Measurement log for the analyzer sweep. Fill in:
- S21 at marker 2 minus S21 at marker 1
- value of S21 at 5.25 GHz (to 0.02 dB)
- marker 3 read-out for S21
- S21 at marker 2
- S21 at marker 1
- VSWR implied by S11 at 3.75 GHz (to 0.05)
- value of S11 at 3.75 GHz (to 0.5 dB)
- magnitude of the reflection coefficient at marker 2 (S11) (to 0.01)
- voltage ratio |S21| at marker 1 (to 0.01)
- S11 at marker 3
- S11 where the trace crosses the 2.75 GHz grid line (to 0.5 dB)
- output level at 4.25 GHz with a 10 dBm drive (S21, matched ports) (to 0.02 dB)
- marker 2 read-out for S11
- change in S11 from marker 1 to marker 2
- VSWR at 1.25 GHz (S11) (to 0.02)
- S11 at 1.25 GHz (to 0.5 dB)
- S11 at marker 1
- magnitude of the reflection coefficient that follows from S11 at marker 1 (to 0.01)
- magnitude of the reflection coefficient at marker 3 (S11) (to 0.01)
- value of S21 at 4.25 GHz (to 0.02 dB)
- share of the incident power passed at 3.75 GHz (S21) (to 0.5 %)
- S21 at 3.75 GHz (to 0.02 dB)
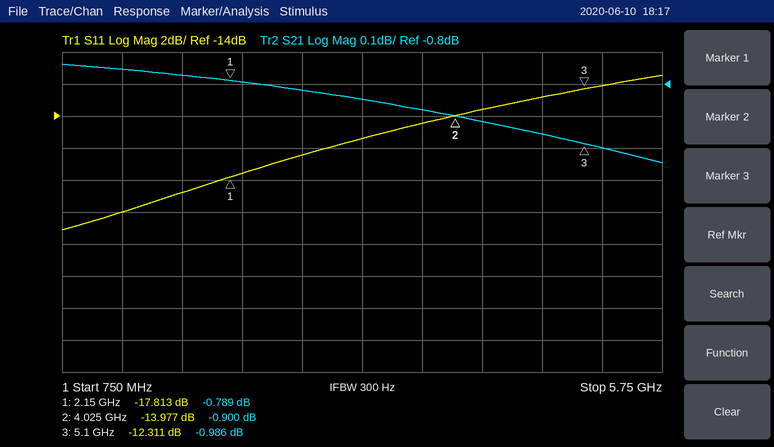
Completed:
-0.111 dB
-1.00 dB
-0.986 dB
-0.900 dB
-0.789 dB
1.45
-14.5 dB
0.20
0.91
-12.311 dB
-16.5 dB
9.08 dBm
-13.977 dB
3.836 dB
1.22
-20.0 dB
-17.813 dB
0.13
0.24
-0.92 dB
81.5 %
-0.88 dB
